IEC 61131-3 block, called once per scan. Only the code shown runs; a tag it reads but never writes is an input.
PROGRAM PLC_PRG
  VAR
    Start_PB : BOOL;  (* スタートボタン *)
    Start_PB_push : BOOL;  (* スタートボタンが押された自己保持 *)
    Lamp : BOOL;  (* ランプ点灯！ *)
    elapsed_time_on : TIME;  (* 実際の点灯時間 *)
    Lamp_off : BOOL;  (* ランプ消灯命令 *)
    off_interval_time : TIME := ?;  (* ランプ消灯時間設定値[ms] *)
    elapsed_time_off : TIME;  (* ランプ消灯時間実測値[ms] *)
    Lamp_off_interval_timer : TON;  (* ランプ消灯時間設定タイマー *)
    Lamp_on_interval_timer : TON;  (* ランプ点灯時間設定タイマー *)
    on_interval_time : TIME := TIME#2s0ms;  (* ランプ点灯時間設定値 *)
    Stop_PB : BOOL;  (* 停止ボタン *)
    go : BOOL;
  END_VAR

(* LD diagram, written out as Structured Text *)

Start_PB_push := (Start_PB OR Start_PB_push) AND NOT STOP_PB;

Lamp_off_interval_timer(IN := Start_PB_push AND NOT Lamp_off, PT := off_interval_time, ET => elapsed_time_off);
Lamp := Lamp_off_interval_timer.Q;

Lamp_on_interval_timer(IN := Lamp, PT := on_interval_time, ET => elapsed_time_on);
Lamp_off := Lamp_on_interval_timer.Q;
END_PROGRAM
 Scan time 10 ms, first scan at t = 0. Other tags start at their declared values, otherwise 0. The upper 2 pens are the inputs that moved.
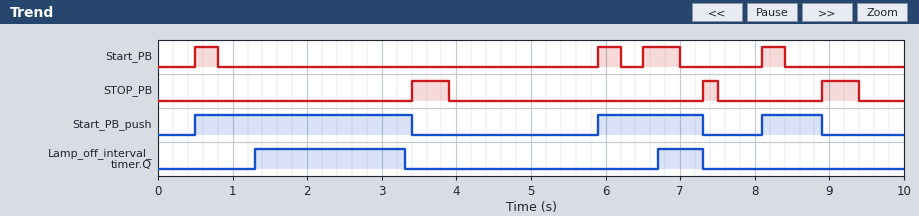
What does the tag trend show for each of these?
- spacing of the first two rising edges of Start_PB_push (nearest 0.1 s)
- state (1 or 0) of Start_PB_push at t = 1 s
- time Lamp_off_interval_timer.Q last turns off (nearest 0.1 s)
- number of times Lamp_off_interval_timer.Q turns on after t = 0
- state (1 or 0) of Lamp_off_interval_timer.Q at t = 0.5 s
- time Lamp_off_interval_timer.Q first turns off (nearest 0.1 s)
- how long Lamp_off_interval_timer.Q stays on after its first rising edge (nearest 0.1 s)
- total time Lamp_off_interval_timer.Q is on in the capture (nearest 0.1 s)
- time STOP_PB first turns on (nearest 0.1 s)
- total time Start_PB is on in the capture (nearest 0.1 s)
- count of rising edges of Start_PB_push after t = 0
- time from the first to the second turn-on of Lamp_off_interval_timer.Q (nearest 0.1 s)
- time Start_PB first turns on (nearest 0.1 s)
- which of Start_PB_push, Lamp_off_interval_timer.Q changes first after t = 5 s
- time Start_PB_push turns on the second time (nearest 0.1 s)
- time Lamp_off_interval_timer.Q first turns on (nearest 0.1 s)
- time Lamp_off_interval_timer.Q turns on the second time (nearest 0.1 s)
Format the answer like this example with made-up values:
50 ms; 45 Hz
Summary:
5.4 s; 1; 7.3 s; 2; 0; 3.3 s; 2.0 s; 2.6 s; 3.4 s; 1.4 s; 3; 5.4 s; 0.5 s; Start_PB_push; 5.9 s; 1.3 s; 6.7 s
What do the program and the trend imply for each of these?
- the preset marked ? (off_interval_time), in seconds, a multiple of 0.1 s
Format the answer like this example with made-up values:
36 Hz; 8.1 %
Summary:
0.8 s
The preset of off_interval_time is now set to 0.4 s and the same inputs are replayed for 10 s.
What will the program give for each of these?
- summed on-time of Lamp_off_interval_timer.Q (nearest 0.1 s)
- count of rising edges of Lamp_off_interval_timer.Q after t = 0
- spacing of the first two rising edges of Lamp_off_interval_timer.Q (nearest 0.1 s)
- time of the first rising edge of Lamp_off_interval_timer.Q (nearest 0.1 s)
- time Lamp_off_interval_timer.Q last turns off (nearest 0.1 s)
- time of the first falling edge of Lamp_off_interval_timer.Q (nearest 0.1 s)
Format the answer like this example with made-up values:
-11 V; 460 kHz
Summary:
3.5 s; 4; 2.4 s; 0.9 s; 8.9 s; 2.9 s
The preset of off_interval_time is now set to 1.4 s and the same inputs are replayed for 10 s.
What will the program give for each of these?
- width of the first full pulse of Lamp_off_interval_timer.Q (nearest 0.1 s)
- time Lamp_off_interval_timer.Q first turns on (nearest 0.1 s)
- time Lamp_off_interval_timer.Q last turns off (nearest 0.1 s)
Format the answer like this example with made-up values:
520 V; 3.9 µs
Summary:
1.5 s; 1.9 s; 3.4 s
